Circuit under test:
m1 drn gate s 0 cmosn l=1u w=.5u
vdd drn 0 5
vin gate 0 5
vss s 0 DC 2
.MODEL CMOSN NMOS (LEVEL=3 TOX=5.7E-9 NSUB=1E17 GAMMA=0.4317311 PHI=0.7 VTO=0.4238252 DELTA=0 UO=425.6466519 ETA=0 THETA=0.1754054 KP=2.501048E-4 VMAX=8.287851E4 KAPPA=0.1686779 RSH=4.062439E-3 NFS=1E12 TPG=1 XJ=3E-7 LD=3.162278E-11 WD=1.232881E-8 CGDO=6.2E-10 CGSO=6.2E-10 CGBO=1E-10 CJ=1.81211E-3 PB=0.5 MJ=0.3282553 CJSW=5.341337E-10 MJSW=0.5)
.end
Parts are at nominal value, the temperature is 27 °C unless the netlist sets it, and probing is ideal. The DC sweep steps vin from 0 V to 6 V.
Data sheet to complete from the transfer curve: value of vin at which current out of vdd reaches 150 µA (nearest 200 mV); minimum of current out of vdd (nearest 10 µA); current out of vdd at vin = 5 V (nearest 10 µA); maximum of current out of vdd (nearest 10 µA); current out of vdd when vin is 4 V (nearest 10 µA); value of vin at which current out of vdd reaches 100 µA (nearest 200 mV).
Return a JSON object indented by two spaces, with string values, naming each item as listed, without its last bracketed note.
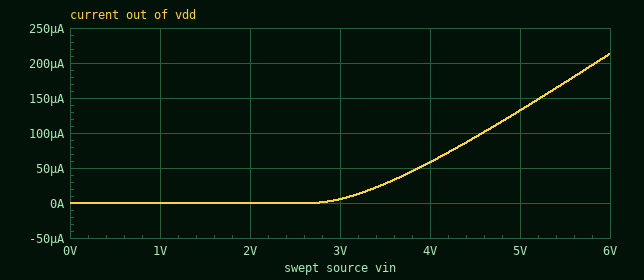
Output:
{
  "value of vin at which current out of vdd reaches 150 µA": "5.2 V",
  "minimum of current out of vdd": "0 A",
  "current out of vdd at vin = 5 V": "130 µA",
  "maximum of current out of vdd": "210 µA",
  "current out of vdd when vin is 4 V": "60 µA",
  "value of vin at which current out of vdd reaches 100 µA": "4.6 V"
}
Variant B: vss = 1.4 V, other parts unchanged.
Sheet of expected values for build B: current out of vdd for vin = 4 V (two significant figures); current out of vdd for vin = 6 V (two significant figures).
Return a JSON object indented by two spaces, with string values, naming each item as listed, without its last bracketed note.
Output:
{
  "current out of vdd for vin = 4 V": "110 µA",
  "current out of vdd for vin = 6 V": "270 µA"
}
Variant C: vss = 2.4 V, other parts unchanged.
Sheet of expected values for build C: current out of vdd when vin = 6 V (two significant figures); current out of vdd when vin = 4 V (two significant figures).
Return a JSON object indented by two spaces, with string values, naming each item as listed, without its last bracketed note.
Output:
{
  "current out of vdd when vin = 6 V": "180 µA",
  "current out of vdd when vin = 4 V": "31 µA"
}
